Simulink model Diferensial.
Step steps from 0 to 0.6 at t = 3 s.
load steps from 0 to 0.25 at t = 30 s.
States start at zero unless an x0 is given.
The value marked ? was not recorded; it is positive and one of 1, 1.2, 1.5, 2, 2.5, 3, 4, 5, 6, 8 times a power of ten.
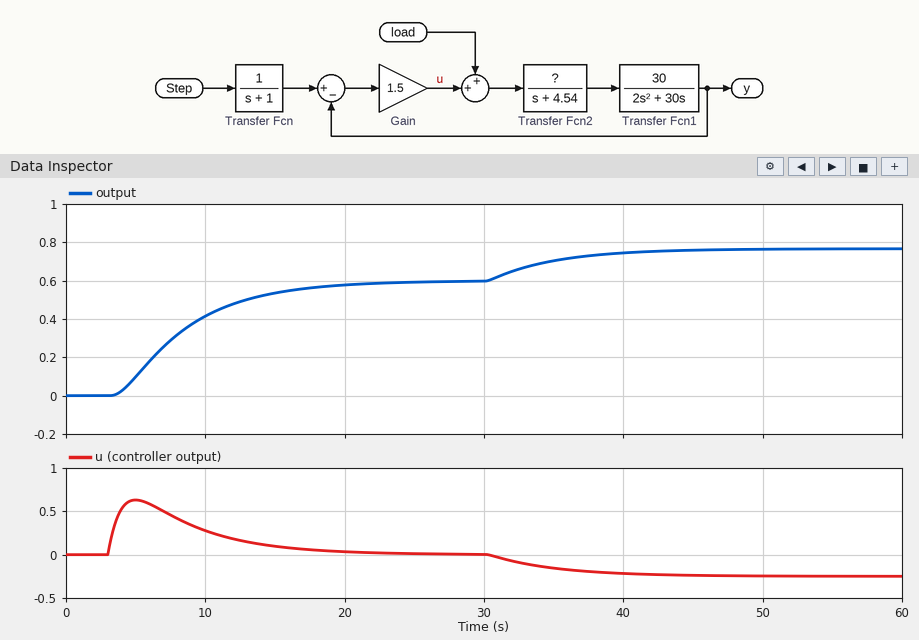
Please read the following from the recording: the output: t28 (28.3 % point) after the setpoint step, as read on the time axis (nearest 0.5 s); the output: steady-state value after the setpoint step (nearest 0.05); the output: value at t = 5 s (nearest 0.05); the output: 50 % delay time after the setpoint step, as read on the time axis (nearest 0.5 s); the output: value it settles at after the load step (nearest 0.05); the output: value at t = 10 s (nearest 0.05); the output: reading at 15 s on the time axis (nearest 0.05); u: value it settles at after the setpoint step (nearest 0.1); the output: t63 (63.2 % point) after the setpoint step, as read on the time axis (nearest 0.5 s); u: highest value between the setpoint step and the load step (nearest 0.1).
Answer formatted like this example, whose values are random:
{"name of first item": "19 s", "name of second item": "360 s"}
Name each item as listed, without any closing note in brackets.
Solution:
{"the output: t28 (28.3 % point) after the setpoint step, as read on the time axis": "6.0 s", "the output: steady-state value after the setpoint step": "0.60", "the output: value at t = 5 s": "0.10", "the output: 50 % delay time after the setpoint step, as read on the time axis": "7.5 s", "the output: value it settles at after the load step": "0.75", "the output: value at t = 10 s": "0.40", "the output: reading at 15 s on the time axis": "0.55", "u: value it settles at after the setpoint step": "0.0", "the output: t63 (63.2 % point) after the setpoint step, as read on the time axis": "9.0 s", "u: highest value between the setpoint step and the load step": "0.6"}
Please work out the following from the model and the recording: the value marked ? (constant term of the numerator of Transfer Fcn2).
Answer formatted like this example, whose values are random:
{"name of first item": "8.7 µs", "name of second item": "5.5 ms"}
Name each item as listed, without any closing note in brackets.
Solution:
{"the value marked ?": "0.6"}
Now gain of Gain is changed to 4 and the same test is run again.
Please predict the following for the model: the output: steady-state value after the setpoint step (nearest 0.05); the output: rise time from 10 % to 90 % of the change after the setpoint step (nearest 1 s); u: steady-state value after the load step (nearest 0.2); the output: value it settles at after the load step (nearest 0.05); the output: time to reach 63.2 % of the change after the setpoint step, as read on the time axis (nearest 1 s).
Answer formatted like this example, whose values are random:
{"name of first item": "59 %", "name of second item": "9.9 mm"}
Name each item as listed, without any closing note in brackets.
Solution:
{"the output: steady-state value after the setpoint step": "0.60", "the output: rise time from 10 % to 90 % of the change after the setpoint step": "4 s", "u: steady-state value after the load step": "-0.2", "the output: value it settles at after the load step": "0.65", "the output: time to reach 63.2 % of the change after the setpoint step, as read on the time axis": "6 s"}
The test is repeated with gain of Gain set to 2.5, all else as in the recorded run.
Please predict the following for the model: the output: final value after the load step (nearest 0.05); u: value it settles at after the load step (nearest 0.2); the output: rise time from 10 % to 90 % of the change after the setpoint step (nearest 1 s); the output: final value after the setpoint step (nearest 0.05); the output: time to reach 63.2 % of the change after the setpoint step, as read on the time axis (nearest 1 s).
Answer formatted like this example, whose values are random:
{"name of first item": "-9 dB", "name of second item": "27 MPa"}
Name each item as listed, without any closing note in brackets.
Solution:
{"the output: final value after the load step": "0.70", "u: value it settles at after the load step": "-0.2", "the output: rise time from 10 % to 90 % of the change after the setpoint step": "7 s", "the output: final value after the setpoint step": "0.60", "the output: time to reach 63.2 % of the change after the setpoint step, as read on the time axis": "7 s"}
